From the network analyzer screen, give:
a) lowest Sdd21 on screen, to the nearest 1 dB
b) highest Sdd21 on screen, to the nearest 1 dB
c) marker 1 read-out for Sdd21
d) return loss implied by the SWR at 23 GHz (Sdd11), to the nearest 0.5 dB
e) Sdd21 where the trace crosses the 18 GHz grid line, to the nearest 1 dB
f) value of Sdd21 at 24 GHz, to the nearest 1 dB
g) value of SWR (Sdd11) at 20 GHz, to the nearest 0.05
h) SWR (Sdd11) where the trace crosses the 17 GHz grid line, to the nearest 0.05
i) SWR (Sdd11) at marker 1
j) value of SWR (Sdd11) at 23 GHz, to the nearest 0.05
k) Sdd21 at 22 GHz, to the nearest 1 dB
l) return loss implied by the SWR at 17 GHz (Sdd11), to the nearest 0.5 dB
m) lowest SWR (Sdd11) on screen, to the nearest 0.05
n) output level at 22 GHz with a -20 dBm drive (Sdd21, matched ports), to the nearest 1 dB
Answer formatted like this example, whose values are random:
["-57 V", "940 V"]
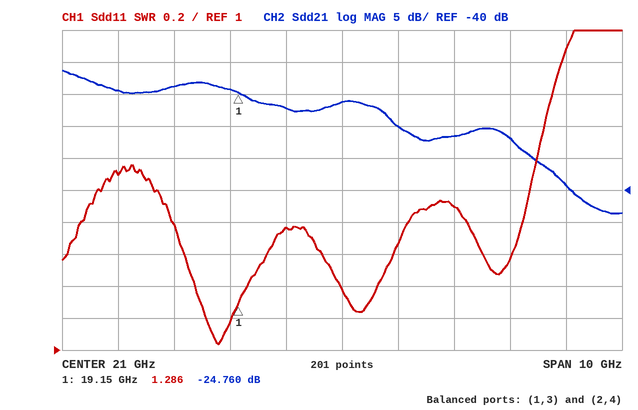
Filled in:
["-44 dB", "-21 dB", "-24.760 dB", "10.0 dB", "-24 dB", "-32 dB", "1.75", "2.10", "1.286", "1.90", "-30 dB", "9.0 dB", "1.05", "-50 dBm"]
